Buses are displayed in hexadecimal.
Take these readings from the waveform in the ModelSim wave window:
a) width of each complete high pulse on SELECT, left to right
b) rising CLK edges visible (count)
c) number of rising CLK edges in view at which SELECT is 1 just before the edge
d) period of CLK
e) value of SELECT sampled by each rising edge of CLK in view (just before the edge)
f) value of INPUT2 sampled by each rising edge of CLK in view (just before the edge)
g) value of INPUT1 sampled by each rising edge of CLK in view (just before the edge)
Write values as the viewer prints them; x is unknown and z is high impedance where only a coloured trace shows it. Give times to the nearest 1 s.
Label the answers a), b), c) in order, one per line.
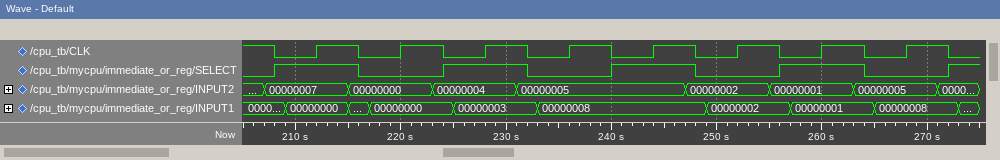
a) 8 s, 8 s, 8 s, 8 s
b) 8
c) 4
d) 8 s
e) 1 0 1 0 1 0 1 0
f) 00000007, 00000000, 00000004, 00000005, 00000005, 00000002, 00000001, 00000005
g) 00000000, 00000000, 00000003, 00000008, 00000008, 00000002, 00000001, 00000008
